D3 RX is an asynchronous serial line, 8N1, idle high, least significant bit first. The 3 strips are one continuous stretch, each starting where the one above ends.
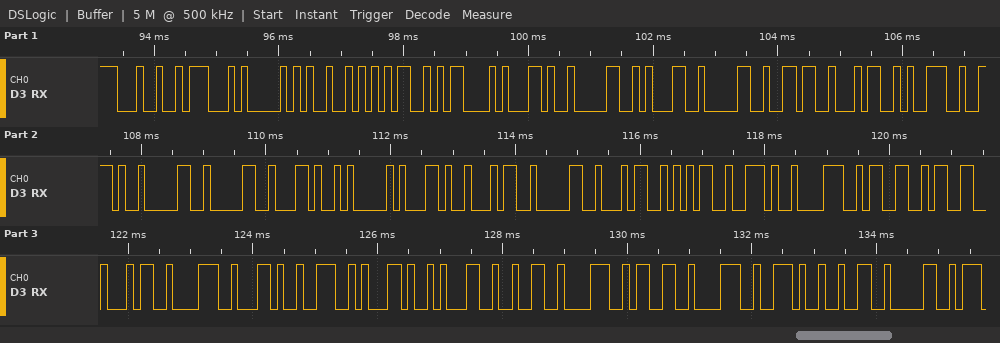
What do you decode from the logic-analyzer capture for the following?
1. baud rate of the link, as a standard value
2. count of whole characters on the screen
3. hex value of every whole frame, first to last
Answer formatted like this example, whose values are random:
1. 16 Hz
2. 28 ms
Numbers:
1. 9600 baud
2. 40
3. 0x24 0x47 0x50 0x52 0x4D 0x43 0x2C 0x30 0x31 0x30 0x36 0x34 0x39 0x2E 0x30 0x30 0x2C 0x41 0x2C 0x34 0x30 0x34 0x35 0x2E 0x38 0x33 0x33 0x34 0x38 0x2C 0x4E 0x2C 0x31 0x32 0x38 0x33 0x38 0x2E 0x32 0x30
